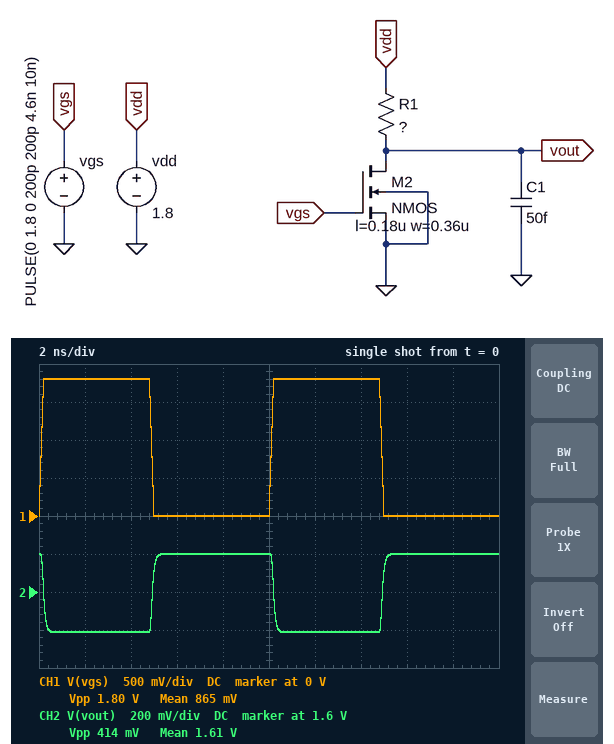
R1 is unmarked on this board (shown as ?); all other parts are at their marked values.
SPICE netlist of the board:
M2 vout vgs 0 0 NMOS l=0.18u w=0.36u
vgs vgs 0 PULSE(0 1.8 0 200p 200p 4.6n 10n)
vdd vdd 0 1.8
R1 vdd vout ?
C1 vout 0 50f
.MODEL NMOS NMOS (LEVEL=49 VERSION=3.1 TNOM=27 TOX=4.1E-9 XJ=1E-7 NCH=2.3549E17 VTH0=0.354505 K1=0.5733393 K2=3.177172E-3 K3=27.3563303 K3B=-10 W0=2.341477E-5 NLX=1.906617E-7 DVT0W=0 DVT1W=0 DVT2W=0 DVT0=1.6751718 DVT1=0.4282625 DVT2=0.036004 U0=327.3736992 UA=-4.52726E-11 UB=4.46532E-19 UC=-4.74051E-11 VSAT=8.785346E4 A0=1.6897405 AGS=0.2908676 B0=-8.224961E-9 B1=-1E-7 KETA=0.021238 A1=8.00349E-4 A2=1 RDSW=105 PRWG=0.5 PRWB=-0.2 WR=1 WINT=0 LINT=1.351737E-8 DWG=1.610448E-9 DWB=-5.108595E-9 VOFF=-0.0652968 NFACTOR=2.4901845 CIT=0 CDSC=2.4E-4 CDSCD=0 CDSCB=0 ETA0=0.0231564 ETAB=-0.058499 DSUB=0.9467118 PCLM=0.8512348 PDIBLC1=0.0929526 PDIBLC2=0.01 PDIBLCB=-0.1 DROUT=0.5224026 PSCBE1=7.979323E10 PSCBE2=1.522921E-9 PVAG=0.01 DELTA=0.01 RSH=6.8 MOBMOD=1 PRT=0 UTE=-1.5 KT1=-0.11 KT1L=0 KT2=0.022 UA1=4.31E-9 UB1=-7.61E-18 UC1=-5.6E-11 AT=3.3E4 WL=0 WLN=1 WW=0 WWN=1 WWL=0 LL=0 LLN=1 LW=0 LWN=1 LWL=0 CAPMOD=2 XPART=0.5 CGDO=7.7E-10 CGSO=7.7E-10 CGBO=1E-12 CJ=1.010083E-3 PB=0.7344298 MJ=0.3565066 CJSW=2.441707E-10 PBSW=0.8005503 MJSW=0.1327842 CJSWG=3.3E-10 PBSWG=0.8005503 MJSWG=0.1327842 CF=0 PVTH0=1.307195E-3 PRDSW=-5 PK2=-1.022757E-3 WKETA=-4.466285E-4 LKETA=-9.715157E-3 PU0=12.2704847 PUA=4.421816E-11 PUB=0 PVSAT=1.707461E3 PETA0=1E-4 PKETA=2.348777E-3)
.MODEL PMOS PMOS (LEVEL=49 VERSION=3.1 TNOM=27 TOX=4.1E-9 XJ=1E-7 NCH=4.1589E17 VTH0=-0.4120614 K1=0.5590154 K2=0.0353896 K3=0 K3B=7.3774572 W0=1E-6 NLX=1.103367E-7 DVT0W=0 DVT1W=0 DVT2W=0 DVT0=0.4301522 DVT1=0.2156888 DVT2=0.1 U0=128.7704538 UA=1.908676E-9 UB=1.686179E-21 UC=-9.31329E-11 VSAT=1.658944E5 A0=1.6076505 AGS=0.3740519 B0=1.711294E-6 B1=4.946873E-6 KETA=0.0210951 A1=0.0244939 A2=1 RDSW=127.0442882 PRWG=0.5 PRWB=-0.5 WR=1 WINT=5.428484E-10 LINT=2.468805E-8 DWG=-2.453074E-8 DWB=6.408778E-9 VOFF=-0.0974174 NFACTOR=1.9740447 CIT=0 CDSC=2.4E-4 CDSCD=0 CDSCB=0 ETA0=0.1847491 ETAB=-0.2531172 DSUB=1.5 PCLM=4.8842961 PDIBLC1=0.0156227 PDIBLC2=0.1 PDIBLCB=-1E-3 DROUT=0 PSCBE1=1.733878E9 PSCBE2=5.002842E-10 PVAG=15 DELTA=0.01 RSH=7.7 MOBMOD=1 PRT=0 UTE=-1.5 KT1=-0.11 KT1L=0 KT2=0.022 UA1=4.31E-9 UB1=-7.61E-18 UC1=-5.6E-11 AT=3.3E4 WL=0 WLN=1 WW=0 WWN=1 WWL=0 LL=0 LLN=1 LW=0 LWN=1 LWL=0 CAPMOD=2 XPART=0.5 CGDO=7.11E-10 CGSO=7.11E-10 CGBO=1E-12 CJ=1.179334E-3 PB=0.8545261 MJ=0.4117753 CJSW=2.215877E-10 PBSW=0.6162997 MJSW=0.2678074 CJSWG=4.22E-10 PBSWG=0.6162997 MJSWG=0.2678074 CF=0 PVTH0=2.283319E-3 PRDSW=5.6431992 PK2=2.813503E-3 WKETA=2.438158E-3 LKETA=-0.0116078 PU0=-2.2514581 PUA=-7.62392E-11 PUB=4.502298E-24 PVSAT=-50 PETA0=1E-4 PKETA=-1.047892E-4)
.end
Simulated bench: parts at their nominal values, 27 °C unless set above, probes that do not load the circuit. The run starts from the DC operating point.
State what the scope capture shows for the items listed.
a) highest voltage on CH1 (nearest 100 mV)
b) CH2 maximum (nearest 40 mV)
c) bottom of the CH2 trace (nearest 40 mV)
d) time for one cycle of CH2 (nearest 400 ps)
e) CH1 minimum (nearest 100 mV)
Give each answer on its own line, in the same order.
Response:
1.8 V
1.80 V
1.40 V
10.0 ns
0 V
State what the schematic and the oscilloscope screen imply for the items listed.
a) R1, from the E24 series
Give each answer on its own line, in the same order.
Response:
1.6 kΩ
